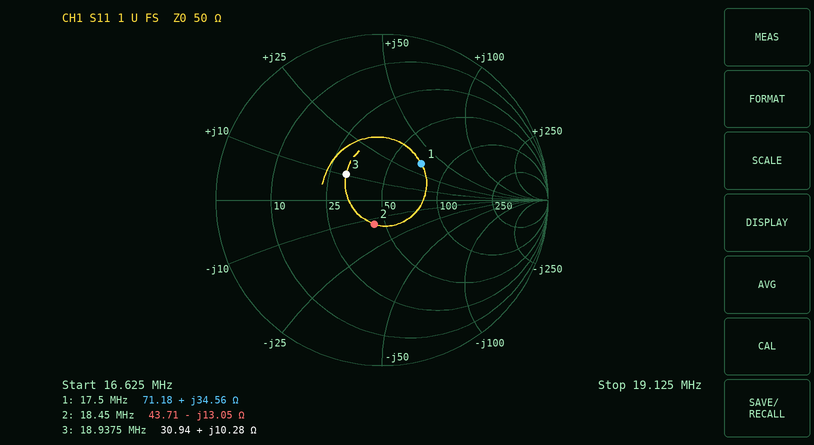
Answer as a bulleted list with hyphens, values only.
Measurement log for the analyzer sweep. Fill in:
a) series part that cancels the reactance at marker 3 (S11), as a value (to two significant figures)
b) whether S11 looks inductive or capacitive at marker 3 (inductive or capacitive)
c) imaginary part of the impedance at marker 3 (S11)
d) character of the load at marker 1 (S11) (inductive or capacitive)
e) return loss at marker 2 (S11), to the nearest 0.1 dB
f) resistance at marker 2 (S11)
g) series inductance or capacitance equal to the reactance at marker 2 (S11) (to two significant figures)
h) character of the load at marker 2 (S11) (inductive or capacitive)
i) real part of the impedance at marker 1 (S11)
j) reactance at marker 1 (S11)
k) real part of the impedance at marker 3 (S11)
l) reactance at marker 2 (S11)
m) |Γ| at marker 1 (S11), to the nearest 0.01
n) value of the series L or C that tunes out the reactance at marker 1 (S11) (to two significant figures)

- 820 pF
- inductive
- +10.28 Ω
- inductive
- 16.3 dB
- 43.71 Ω
- 660 pF
- capacitive
- 71.18 Ω
- +34.56 Ω
- 30.94 Ω
- -13.05 Ω
- 0.32
- 260 pF
